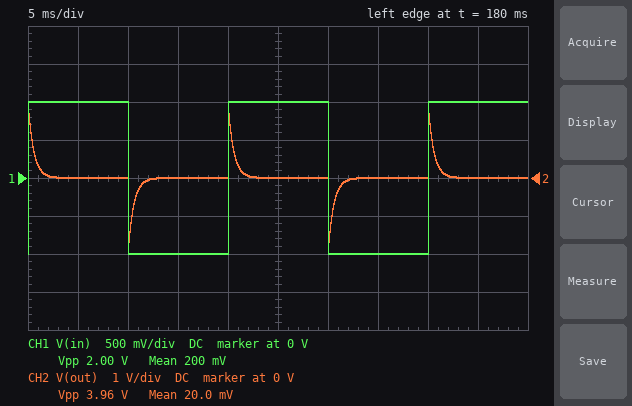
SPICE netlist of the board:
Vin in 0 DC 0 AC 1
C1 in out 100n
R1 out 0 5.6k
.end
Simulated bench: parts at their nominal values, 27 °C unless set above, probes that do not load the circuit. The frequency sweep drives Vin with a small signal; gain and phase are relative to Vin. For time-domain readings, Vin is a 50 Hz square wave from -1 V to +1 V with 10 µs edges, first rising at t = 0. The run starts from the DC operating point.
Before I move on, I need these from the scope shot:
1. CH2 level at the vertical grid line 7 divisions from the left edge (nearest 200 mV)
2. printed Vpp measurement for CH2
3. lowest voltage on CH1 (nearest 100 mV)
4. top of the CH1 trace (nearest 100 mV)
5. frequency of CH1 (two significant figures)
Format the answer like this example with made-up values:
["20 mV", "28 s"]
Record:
["0 V", "3.96 V", "-1.0 V", "1.0 V", "50 Hz"]
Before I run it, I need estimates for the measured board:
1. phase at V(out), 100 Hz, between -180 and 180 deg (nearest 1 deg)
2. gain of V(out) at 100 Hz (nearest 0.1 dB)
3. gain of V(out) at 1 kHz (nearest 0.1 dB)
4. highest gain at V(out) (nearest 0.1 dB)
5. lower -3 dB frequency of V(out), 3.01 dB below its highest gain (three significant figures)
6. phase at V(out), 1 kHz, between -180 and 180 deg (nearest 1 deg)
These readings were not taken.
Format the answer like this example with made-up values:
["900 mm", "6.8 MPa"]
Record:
["71 deg", "-9.6 dB", "-0.3 dB", "0 dB", "284 Hz", "16 deg"]
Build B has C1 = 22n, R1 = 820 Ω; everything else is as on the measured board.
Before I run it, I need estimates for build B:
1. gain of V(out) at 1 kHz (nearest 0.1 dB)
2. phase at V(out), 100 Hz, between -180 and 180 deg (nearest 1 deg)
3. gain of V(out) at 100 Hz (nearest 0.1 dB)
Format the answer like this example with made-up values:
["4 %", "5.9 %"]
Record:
["-19.0 dB", "89 deg", "-38.9 dB"]
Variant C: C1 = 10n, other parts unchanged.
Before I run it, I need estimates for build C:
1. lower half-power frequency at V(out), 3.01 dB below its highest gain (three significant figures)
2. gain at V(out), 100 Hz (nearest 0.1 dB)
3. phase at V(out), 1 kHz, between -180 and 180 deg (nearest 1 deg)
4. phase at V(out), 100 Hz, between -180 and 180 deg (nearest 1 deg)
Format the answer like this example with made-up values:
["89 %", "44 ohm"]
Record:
["2.84 kHz", "-29.1 dB", "71 deg", "88 deg"]
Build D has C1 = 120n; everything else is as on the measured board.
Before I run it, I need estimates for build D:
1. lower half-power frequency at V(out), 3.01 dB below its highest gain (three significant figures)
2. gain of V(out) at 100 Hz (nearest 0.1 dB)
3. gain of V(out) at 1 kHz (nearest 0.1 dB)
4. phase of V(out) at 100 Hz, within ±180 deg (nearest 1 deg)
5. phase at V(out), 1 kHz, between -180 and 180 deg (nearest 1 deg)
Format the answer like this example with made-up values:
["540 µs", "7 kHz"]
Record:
["237 Hz", "-8.2 dB", "-0.2 dB", "67 deg", "13 deg"]
